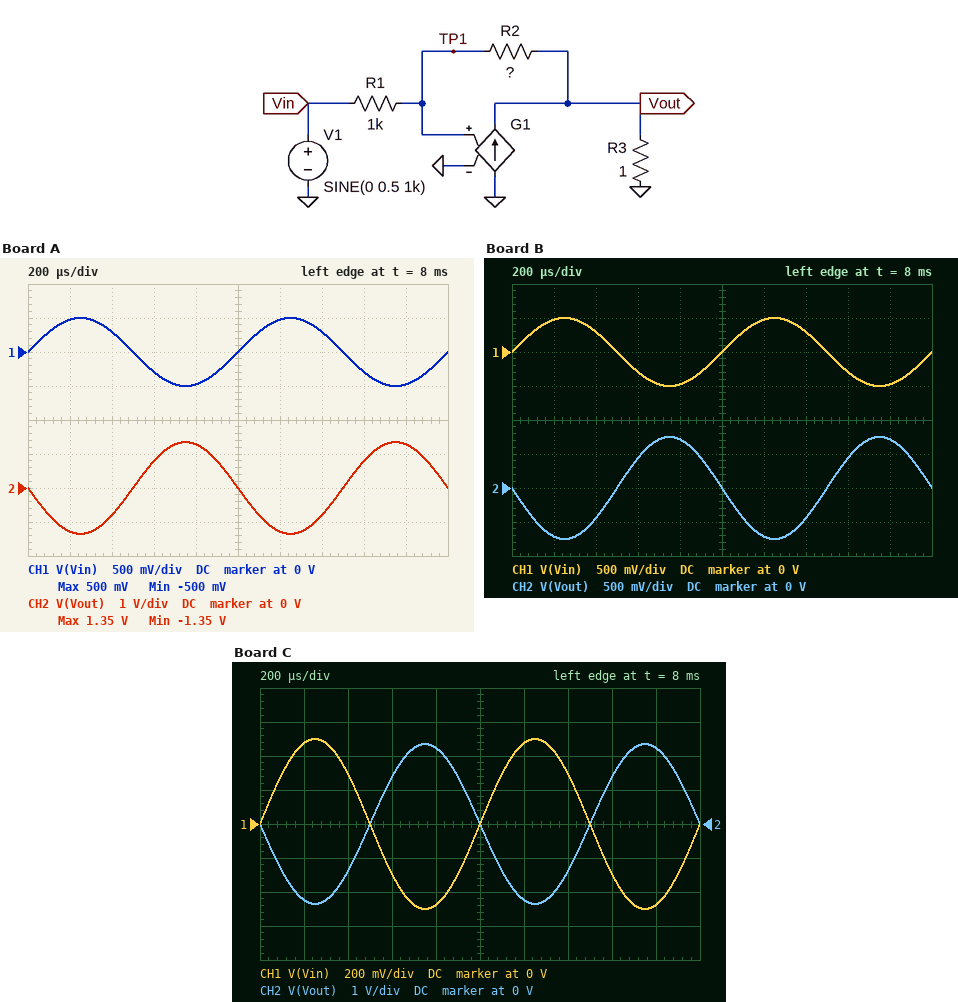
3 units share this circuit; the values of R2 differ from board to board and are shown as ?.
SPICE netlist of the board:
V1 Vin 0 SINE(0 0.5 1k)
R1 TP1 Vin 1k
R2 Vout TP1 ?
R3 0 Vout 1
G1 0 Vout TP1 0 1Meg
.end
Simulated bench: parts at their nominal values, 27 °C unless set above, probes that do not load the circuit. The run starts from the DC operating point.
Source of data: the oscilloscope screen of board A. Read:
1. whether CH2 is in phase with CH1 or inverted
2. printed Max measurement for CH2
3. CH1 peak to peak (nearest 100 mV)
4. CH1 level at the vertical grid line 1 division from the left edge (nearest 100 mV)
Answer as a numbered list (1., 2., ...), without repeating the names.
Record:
1. inverted
2. 1.35 V
3. 1.0 V
4. 500 mV
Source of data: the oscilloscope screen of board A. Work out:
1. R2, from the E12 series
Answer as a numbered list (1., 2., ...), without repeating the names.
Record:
1. 2.7 kΩ
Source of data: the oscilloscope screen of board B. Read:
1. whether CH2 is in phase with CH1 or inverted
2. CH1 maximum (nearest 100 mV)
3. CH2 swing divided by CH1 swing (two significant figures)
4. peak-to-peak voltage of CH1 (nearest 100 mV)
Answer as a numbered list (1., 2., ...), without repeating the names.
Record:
1. inverted
2. 500 mV
3. 1.5
4. 1.0 V
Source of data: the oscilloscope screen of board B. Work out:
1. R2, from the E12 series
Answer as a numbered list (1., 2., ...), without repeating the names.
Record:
1. 1.5 kΩ
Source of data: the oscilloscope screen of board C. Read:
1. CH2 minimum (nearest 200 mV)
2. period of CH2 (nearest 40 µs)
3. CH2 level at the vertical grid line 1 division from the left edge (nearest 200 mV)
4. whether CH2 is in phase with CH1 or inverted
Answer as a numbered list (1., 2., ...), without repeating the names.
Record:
1. -2.4 V
2. 1.00 ms
3. -2.2 V
4. inverted
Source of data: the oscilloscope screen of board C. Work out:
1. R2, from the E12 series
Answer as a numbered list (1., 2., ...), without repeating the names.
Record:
1. 4.7 kΩ
